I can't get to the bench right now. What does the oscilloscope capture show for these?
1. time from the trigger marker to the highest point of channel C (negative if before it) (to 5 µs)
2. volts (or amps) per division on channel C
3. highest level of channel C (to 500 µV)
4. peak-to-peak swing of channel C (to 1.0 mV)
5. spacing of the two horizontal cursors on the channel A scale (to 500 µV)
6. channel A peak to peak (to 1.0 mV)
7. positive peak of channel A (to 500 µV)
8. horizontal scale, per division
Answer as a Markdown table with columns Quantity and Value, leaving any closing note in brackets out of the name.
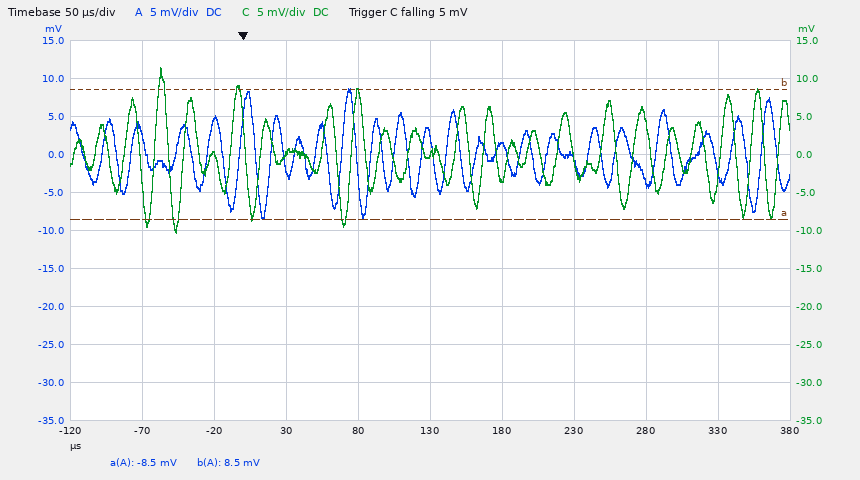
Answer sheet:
| Quantity | Value |
|---|---|
| time from the trigger marker to the highest point of channel C (negative if before it) | -55 µs |
| volts (or amps) per division on channel C | 5 mV |
| highest level of channel C | 11.5 mV |
| peak-to-peak swing of channel C | 22.0 mV |
| spacing of the two horizontal cursors on the channel A scale | 17.0 mV |
| channel A peak to peak | 17.0 mV |
| positive peak of channel A | 8.5 mV |
| horizontal scale, per division | 50 µs |
